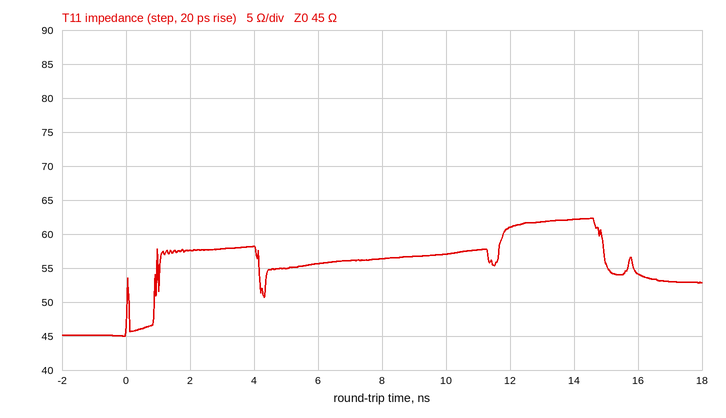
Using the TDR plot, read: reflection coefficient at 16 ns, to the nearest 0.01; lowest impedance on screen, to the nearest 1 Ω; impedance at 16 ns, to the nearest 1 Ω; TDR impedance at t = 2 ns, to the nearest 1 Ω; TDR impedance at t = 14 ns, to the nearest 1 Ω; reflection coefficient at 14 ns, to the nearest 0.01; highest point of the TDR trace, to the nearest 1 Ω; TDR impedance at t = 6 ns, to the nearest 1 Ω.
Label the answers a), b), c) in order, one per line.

a) +0.09
b) 45 Ω
c) 54 Ω
d) 58 Ω
e) 62 Ω
f) +0.16
g) 62 Ω
h) 56 Ω
